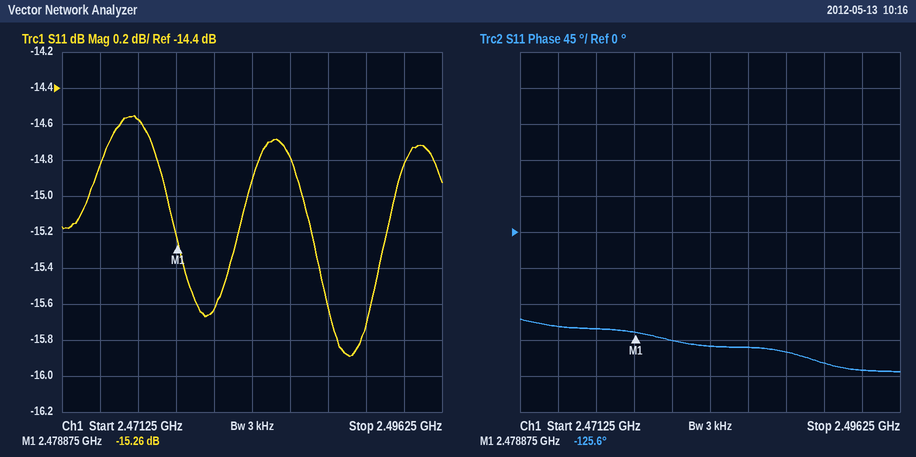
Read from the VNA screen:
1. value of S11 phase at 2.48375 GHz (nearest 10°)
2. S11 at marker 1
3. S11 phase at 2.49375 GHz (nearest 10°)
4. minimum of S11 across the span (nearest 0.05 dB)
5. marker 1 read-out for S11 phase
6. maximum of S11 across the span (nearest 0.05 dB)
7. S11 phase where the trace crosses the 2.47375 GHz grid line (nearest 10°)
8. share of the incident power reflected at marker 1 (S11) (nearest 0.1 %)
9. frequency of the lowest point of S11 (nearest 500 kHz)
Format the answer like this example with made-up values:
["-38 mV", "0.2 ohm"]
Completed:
["-140°", "-15.26 dB", "-170°", "-15.90 dB", "-125.6°", "-14.55 dB", "-120°", "3.0 %", "2.4900 GHz"]
